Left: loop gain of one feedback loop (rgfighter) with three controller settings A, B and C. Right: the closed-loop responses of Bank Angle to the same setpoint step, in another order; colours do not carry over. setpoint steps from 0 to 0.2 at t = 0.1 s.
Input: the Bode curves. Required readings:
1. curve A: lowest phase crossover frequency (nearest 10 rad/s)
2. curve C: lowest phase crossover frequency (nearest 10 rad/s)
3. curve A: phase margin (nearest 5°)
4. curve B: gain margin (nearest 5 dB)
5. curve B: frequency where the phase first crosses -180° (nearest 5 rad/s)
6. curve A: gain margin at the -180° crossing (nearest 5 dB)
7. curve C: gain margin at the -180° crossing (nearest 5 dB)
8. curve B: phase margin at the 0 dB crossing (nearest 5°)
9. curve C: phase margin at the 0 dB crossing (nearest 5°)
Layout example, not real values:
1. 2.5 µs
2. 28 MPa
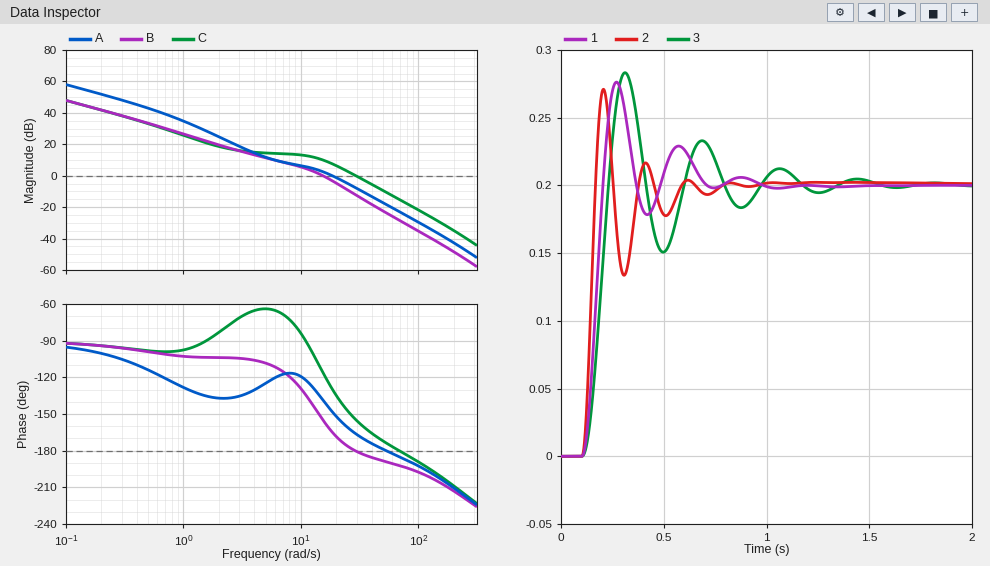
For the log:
1. 50 rad/s
2. 70 rad/s
3. 30°
4. 10 dB
5. 30 rad/s
6. 20 dB
7. 15 dB
8. 25°
9. 25°
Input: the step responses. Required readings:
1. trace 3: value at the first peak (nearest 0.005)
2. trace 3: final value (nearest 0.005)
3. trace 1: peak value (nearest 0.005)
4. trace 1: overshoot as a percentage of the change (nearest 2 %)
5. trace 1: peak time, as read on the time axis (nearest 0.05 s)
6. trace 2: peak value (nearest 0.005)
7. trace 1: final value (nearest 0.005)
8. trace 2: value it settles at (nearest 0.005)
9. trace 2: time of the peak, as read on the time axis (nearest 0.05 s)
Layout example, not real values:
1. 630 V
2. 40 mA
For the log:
1. 0.285
2. 0.200
3. 0.275
4. 38 %
5. 0.25 s
6. 0.270
7. 0.200
8. 0.200
9. 0.20 s
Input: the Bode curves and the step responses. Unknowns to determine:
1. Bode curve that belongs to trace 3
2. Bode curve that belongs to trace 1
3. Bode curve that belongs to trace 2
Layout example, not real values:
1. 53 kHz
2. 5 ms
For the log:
1. B
2. A
3. C
